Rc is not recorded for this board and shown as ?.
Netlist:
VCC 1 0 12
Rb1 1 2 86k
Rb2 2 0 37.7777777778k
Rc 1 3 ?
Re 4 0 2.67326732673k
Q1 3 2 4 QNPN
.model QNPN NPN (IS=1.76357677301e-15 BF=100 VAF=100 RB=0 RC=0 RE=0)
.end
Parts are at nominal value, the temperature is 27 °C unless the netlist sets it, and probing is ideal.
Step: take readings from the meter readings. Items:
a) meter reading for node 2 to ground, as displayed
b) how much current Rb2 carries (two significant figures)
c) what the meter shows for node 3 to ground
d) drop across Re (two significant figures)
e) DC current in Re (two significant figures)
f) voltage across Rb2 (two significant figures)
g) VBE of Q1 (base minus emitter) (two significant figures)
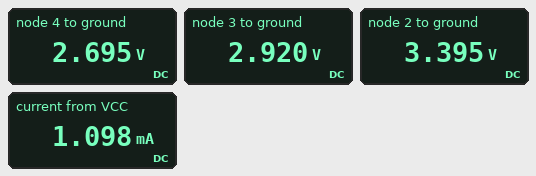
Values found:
3.395 V
90 µA
2.920 V
2.7 V
1.0 mA
3.4 V
700 mV
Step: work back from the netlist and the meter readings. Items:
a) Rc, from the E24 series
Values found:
9.1 kΩ
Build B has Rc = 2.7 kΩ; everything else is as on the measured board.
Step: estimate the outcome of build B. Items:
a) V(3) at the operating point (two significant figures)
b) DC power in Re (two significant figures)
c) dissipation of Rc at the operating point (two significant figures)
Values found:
9.3 V
2.8 mW
2.7 mW
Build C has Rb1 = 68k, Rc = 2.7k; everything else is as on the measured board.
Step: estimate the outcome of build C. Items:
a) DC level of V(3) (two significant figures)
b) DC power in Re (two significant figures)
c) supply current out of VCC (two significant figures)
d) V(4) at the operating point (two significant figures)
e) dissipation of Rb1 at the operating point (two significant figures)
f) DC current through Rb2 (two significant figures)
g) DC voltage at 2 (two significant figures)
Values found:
8.7 V
4.1 mW
1.3 mA
3.3 V
940 µW
110 µA
4.0 V
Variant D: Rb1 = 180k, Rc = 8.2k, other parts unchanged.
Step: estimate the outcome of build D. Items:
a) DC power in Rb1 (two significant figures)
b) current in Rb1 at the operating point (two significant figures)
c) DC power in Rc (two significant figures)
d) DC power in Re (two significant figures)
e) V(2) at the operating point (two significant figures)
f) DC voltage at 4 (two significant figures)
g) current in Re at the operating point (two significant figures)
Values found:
560 µW
56 µA
1.8 mW
600 µW
1.9 V
1.3 V
470 µA
